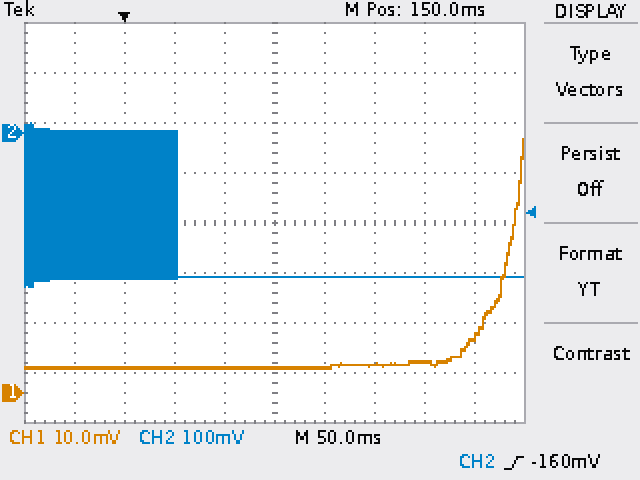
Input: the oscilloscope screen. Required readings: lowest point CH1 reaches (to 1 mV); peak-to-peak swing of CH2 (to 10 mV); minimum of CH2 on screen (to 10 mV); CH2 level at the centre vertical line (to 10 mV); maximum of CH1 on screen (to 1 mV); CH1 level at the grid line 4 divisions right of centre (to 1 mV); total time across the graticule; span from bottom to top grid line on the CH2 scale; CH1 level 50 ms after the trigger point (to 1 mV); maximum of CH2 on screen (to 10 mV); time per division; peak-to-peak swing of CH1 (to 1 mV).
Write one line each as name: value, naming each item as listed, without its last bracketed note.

lowest point CH1 reaches: 5 mV
peak-to-peak swing of CH2: 330 mV
minimum of CH2 on screen: -310 mV
CH2 level at the centre vertical line: -290 mV
maximum of CH1 on screen: 51 mV
CH1 level at the grid line 4 divisions right of centre: 11 mV
total time across the graticule: 500 ms
span from bottom to top grid line on the CH2 scale: 800 mV
CH1 level 50 ms after the trigger point: 5 mV
maximum of CH2 on screen: 20 mV
time per division: 50 ms
peak-to-peak swing of CH1: 46 mV
